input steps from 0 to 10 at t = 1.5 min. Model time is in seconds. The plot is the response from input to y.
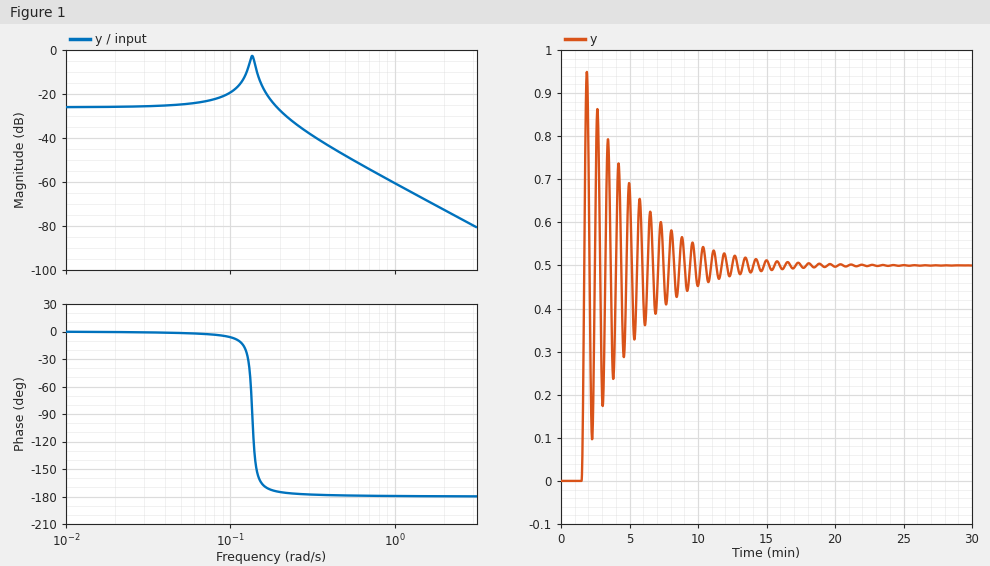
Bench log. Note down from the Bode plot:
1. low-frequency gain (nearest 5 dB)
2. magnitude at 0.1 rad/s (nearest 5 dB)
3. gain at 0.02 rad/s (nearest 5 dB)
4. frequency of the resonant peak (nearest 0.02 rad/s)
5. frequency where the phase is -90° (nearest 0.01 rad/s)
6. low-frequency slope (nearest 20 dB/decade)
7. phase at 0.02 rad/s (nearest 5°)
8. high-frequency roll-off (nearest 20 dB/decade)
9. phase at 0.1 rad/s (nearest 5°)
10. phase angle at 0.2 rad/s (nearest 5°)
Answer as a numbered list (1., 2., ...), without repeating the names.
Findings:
1. -25 dB
2. -20 dB
3. -25 dB
4. 0.14 rad/s
5. 0.14 rad/s
6. 0 dB/decade
7. 0°
8. -40 dB/decade
9. -5°
10. -175°
